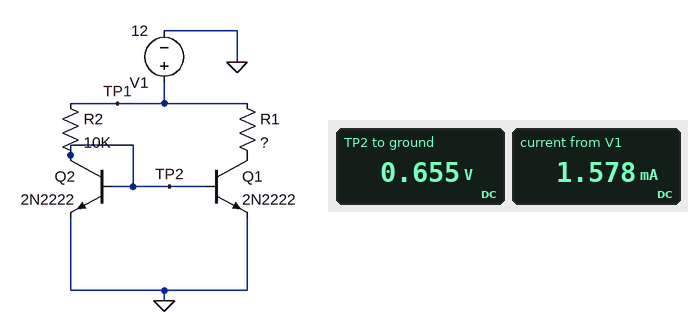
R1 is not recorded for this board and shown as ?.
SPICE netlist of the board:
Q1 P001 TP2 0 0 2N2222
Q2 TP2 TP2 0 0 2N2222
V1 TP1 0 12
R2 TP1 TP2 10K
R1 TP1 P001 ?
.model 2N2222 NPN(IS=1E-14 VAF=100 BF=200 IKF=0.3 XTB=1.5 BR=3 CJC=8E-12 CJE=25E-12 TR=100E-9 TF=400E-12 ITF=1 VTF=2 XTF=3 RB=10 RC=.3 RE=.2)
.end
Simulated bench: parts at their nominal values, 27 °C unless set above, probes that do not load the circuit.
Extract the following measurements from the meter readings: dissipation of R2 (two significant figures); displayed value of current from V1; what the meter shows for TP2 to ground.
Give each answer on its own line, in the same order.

13 mW
1.578 mA
0.655 V
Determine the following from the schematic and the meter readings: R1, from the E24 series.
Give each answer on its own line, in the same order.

27 kΩ
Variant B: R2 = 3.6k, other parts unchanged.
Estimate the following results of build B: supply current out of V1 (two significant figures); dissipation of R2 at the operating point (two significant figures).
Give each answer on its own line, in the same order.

3.6 mA
36 mW
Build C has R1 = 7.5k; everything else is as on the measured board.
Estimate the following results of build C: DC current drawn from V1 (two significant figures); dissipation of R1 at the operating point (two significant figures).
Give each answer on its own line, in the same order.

2.3 mA
10 mW
